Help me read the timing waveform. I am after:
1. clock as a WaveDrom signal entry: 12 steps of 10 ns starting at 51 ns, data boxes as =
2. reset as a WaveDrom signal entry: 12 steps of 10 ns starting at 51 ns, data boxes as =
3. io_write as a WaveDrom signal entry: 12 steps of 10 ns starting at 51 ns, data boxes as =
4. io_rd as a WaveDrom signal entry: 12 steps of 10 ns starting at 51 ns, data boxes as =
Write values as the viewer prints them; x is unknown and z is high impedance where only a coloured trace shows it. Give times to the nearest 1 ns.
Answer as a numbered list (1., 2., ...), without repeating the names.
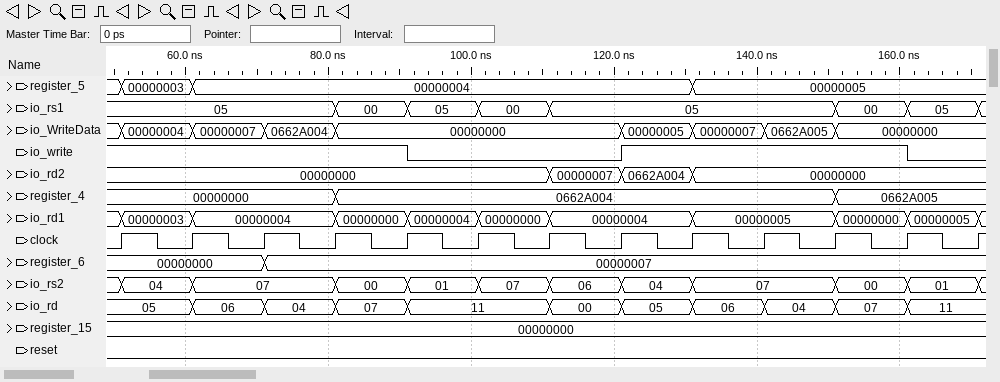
1. {name: 'clock', wave: 'p...........'}
2. {name: 'reset', wave: '0...........'}
3. {name: 'io_write', wave: '1...0..1...0'}
4. {name: 'io_rd', wave: '=====.======', data: '05 06 04 07 11 00 05 06 04 07 11'}
